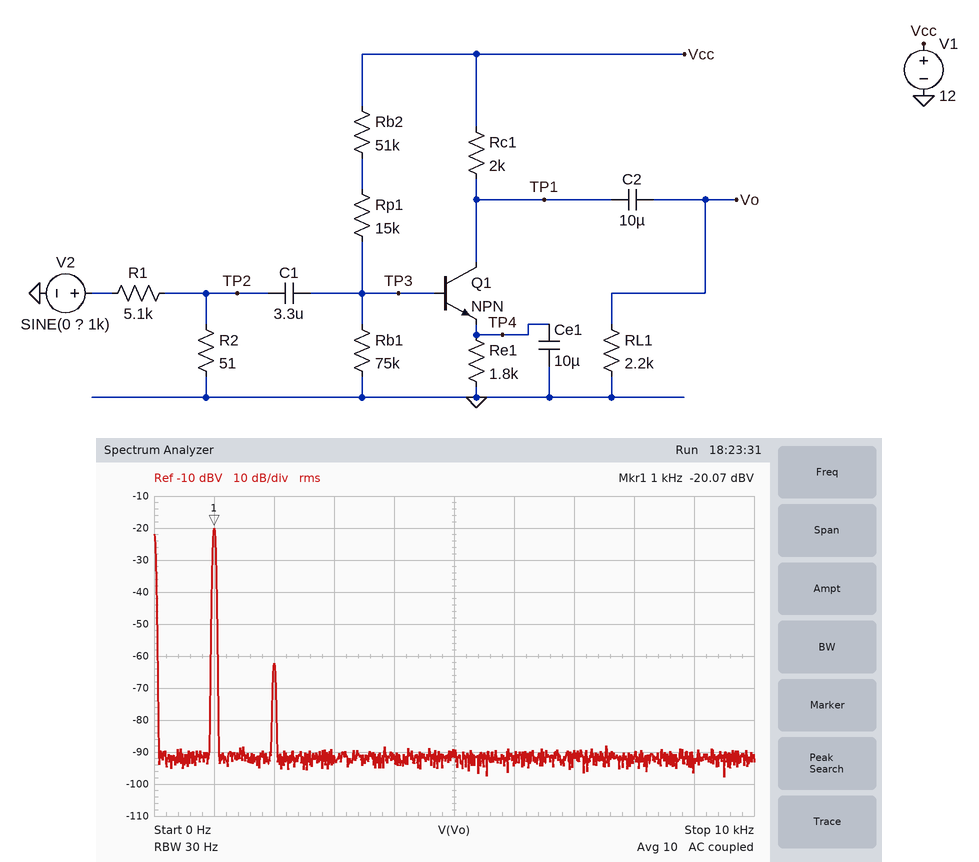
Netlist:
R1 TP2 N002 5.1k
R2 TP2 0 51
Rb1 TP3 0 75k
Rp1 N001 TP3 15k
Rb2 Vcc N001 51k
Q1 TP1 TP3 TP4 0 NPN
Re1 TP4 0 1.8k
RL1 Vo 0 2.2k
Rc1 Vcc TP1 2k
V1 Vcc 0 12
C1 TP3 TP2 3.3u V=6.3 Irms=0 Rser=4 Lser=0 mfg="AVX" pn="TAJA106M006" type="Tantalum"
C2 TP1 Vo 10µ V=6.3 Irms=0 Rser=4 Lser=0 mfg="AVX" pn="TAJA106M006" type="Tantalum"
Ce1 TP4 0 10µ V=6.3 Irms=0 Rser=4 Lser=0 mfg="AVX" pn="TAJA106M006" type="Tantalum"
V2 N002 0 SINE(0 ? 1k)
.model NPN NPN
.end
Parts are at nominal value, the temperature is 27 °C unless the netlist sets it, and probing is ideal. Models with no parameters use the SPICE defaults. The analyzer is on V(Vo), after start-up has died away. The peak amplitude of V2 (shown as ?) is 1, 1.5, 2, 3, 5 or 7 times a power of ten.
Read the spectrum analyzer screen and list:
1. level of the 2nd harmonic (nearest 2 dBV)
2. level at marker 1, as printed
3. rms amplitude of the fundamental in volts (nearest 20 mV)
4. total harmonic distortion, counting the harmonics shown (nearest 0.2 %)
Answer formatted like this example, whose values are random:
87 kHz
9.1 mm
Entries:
-62 dBV
-20.07 dBV
100 mV
0.8 %
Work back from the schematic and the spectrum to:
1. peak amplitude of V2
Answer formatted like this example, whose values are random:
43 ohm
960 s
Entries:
300 mV
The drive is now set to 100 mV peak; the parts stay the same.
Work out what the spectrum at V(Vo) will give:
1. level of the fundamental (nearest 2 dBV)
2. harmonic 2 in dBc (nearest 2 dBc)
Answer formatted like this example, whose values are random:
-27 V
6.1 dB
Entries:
-30 dBV
-52 dBc
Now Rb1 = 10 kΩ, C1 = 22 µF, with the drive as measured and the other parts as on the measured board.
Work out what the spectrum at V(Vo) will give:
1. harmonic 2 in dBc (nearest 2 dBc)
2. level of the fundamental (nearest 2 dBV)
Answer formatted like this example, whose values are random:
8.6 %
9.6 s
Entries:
-32 dBc
-30 dBV
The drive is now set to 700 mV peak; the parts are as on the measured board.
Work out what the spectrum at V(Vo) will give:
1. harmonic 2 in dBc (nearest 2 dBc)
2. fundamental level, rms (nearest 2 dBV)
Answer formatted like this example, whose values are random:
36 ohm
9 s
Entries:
-34 dBc
-12 dBV
